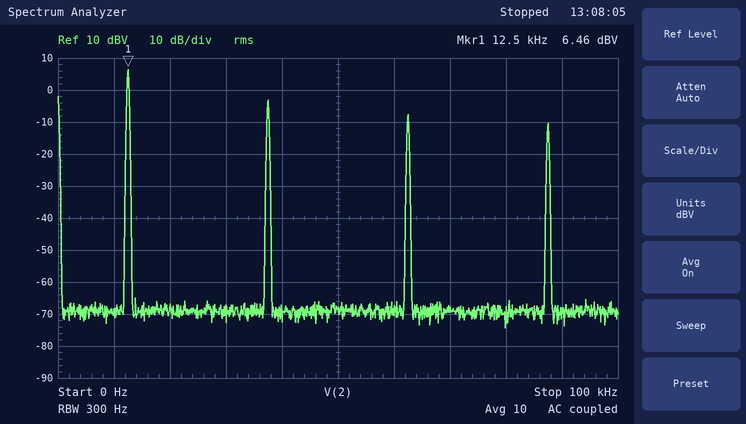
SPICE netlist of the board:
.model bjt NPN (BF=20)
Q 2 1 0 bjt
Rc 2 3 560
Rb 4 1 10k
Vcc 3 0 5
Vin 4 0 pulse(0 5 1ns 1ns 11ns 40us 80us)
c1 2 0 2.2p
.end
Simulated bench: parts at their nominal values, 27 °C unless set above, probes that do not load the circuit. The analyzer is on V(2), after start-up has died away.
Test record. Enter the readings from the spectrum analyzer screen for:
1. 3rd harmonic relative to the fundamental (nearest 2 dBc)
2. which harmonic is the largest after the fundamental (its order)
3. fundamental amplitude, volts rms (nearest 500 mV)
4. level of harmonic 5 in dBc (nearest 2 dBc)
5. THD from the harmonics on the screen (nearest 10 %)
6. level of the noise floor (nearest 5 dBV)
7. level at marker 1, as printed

-10 dBc
3
2.0 V
-14 dBc
40 %
-70 dBV
6.46 dBV
